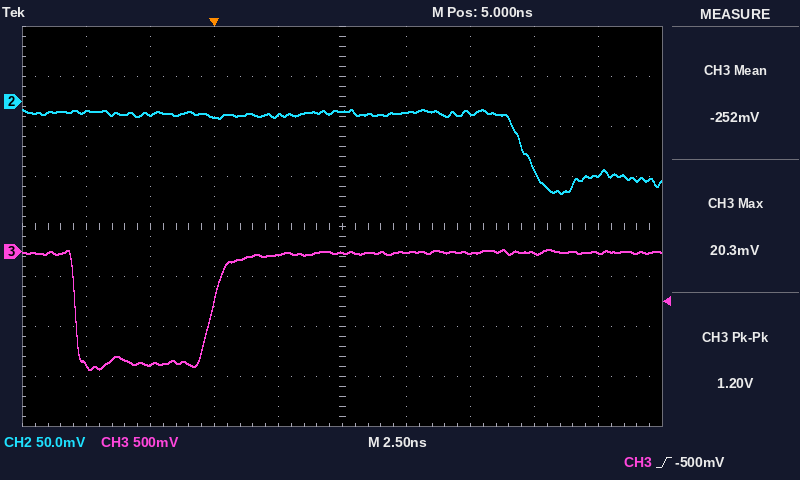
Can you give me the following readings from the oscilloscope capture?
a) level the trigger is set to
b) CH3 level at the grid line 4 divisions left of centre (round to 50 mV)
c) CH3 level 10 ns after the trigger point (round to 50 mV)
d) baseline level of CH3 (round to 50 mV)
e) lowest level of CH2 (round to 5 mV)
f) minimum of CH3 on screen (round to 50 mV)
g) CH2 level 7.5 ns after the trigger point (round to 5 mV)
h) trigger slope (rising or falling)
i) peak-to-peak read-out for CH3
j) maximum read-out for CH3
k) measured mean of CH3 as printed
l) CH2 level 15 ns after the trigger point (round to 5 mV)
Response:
-500 mV
-1.15 V
0 mV
0 mV
-90 mV
-1.20 V
-10 mV
rising
1.20 V
20.3 mV
-252 mV
-75 mV
